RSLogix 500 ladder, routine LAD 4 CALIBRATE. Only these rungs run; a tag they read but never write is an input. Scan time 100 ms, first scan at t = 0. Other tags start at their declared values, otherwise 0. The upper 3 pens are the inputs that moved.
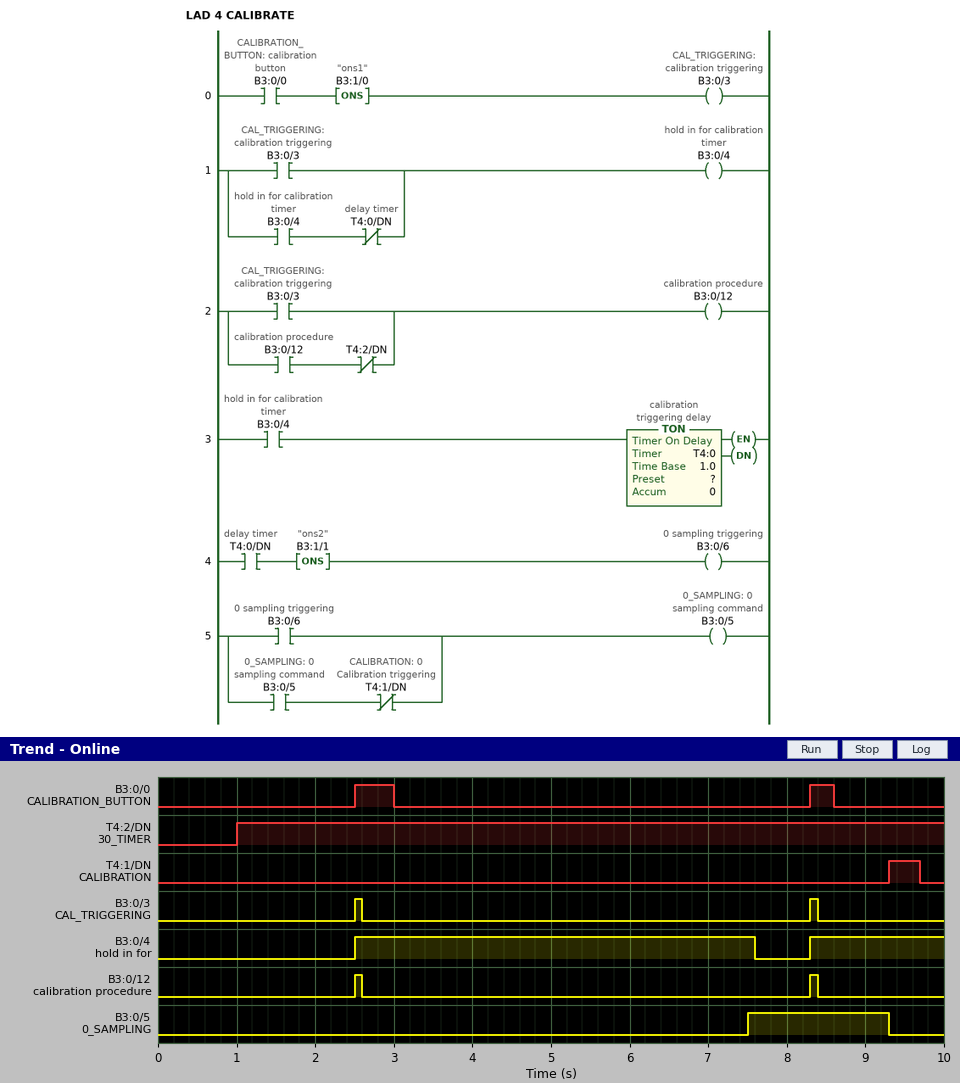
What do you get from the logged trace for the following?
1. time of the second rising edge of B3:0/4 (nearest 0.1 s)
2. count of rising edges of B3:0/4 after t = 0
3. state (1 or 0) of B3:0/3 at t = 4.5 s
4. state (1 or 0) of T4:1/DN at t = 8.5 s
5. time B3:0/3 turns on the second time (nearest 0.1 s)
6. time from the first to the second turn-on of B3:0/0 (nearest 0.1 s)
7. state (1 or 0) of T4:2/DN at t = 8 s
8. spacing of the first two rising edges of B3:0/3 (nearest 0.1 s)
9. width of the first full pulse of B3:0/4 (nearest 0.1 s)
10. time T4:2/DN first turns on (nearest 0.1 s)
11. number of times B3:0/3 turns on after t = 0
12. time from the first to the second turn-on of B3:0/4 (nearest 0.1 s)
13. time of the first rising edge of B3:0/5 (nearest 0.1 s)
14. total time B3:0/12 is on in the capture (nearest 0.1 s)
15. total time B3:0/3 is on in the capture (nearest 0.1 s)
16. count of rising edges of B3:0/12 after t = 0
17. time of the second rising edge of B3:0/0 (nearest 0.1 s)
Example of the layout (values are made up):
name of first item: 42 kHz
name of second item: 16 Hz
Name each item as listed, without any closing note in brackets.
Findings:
time of the second rising edge of B3:0/4: 8.3 s
count of rising edges of B3:0/4 after t = 0: 2
state (1 or 0) of B3:0/3 at t = 4.5 s: 0
state (1 or 0) of T4:1/DN at t = 8.5 s: 0
time B3:0/3 turns on the second time: 8.3 s
time from the first to the second turn-on of B3:0/0: 5.8 s
state (1 or 0) of T4:2/DN at t = 8 s: 1
spacing of the first two rising edges of B3:0/3: 5.8 s
width of the first full pulse of B3:0/4: 5.1 s
time T4:2/DN first turns on: 1.0 s
number of times B3:0/3 turns on after t = 0: 2
time from the first to the second turn-on of B3:0/4: 5.8 s
time of the first rising edge of B3:0/5: 7.5 s
total time B3:0/12 is on in the capture: 0.2 s
total time B3:0/3 is on in the capture: 0.2 s
count of rising edges of B3:0/12 after t = 0: 2
time of the second rising edge of B3:0/0: 8.3 s
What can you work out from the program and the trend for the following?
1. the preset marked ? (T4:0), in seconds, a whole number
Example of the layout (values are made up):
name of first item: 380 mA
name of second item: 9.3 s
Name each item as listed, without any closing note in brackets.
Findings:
the preset marked ? (T4:0), in seconds, a whole number: 5 s
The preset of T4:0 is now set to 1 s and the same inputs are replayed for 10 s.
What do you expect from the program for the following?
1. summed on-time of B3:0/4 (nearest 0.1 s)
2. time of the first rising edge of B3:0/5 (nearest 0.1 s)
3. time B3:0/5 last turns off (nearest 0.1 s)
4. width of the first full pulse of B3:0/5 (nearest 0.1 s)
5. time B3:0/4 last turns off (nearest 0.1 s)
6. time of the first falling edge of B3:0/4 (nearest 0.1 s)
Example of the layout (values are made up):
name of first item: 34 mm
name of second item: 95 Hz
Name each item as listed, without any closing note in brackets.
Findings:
summed on-time of B3:0/4: 2.2 s
time of the first rising edge of B3:0/5: 3.5 s
time B3:0/5 last turns off: 9.4 s
width of the first full pulse of B3:0/5: 5.9 s
time B3:0/4 last turns off: 9.4 s
time of the first falling edge of B3:0/4: 3.6 s
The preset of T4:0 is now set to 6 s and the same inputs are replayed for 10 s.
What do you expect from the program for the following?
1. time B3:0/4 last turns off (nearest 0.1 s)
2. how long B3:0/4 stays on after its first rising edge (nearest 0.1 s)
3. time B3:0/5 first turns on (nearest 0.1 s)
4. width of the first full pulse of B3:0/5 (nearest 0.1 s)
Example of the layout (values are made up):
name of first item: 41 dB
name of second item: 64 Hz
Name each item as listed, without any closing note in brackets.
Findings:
time B3:0/4 last turns off: 8.6 s
how long B3:0/4 stays on after its first rising edge: 6.1 s
time B3:0/5 first turns on: 8.5 s
width of the first full pulse of B3:0/5: 0.8 s
